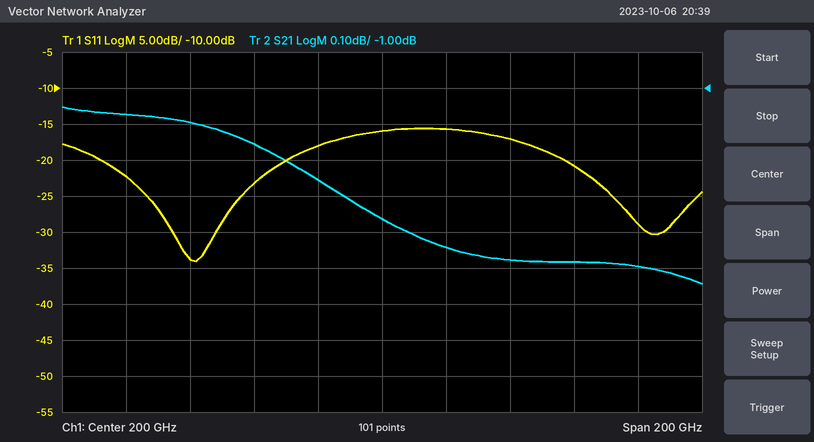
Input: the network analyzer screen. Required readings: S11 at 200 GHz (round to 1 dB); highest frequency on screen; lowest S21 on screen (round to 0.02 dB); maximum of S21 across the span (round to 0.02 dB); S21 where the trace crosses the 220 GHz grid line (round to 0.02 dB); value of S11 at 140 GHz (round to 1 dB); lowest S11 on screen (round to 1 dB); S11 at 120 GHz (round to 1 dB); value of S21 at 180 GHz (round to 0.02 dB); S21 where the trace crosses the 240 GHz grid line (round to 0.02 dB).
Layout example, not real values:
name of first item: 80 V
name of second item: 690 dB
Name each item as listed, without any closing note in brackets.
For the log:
S11 at 200 GHz: -16 dB
highest frequency on screen: 300 GHz
lowest S21 on screen: -1.54 dB
maximum of S21 across the span: -1.06 dB
S21 where the trace crosses the 220 GHz grid line: -1.44 dB
value of S11 at 140 GHz: -34 dB
lowest S11 on screen: -34 dB
S11 at 120 GHz: -22 dB
value of S21 at 180 GHz: -1.26 dB
S21 where the trace crosses the 240 GHz grid line: -1.48 dB
